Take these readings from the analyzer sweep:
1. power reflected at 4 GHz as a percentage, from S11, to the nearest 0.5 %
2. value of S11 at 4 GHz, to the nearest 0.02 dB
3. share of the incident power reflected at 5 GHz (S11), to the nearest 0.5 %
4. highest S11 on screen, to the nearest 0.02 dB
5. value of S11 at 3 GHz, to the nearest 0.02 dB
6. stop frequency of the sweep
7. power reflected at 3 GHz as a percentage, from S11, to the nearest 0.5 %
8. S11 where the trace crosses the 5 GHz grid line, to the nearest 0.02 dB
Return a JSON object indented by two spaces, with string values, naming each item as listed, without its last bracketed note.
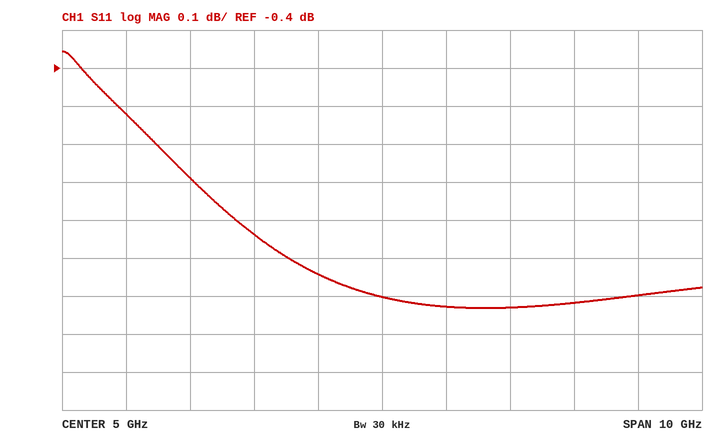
{
  "power reflected at 4 GHz as a percentage, from S11, to the nearest 0.5 %": "80.5 %",
  "value of S11 at 4 GHz, to the nearest 0.02 dB": "-0.94 dB",
  "share of the incident power reflected at 5 GHz (S11), to the nearest 0.5 %": "79.5 %",
  "highest S11 on screen, to the nearest 0.02 dB": "-0.36 dB",
  "value of S11 at 3 GHz, to the nearest 0.02 dB": "-0.84 dB",
  "stop frequency of the sweep": "10 GHz",
  "power reflected at 3 GHz as a percentage, from S11, to the nearest 0.5 %": "82.5 %",
  "S11 where the trace crosses the 5 GHz grid line, to the nearest 0.02 dB": "-1.00 dB"
}
